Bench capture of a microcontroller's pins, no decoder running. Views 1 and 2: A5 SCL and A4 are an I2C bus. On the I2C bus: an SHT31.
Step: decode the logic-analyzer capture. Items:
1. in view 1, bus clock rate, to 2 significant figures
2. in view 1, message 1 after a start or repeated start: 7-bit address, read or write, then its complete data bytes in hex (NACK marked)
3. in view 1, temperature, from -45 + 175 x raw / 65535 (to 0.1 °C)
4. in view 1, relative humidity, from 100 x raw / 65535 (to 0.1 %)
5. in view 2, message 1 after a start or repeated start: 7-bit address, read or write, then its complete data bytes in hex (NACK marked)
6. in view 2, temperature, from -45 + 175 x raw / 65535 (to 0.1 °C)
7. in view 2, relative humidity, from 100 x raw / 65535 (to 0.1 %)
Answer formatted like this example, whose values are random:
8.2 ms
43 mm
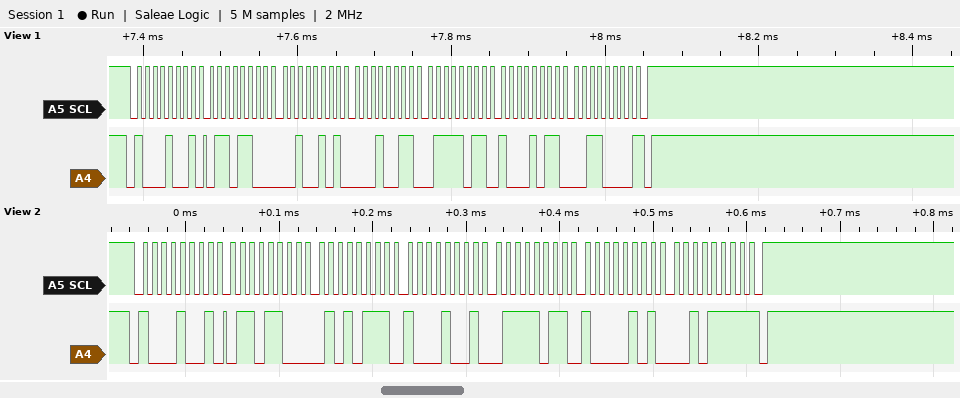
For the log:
100 kHz
0x44 read: 6C 25 13 7B 8B 30 NACK
28.9 °C
48.3 %
0x44 read: 6C 57 89 7B 85 2F NACK
29.1 °C
48.3 %
